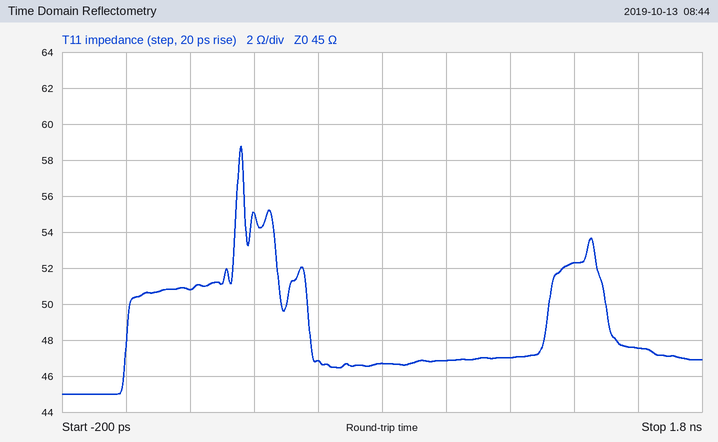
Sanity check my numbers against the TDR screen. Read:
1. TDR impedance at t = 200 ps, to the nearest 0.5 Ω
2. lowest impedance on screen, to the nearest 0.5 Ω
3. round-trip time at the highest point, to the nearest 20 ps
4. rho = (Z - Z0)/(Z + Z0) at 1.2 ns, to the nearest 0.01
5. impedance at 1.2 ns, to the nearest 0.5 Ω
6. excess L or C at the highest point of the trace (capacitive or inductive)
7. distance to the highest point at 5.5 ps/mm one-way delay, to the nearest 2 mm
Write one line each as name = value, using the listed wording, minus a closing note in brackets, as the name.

TDR impedance at t = 200 ps, to the nearest 0.5 Ω = 51.0 Ω
lowest impedance on screen, to the nearest 0.5 Ω = 45.0 Ω
round-trip time at the highest point, to the nearest 20 ps = 360 ps
rho = (Z - Z0)/(Z + Z0) at 1.2 ns, to the nearest 0.01 = +0.02
impedance at 1.2 ns, to the nearest 0.5 Ω = 47.0 Ω
excess L or C at the highest point of the trace = inductive
distance to the highest point at 5.5 ps/mm one-way delay, to the nearest 2 mm = 32 mm
